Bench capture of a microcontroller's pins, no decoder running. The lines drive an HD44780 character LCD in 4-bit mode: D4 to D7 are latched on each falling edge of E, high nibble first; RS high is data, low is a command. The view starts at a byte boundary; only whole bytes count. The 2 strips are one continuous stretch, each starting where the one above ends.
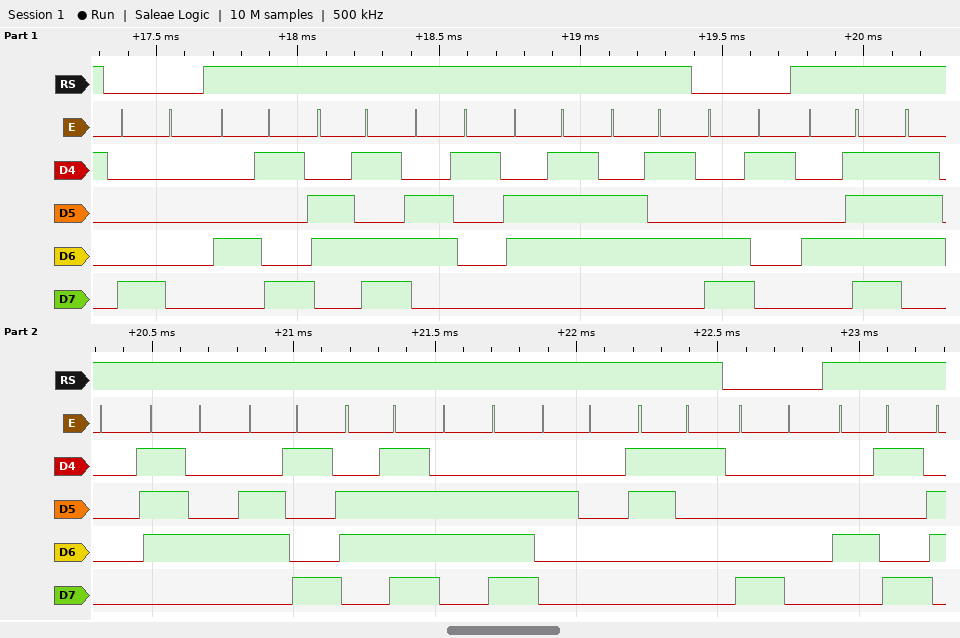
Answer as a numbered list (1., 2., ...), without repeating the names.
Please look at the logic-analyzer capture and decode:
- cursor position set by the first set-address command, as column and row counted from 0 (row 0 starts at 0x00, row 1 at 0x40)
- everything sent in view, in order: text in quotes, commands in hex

1. column 0, row 0
2. 0x80 "Image" 0xC1 "Option 1" 0x80 "I"
